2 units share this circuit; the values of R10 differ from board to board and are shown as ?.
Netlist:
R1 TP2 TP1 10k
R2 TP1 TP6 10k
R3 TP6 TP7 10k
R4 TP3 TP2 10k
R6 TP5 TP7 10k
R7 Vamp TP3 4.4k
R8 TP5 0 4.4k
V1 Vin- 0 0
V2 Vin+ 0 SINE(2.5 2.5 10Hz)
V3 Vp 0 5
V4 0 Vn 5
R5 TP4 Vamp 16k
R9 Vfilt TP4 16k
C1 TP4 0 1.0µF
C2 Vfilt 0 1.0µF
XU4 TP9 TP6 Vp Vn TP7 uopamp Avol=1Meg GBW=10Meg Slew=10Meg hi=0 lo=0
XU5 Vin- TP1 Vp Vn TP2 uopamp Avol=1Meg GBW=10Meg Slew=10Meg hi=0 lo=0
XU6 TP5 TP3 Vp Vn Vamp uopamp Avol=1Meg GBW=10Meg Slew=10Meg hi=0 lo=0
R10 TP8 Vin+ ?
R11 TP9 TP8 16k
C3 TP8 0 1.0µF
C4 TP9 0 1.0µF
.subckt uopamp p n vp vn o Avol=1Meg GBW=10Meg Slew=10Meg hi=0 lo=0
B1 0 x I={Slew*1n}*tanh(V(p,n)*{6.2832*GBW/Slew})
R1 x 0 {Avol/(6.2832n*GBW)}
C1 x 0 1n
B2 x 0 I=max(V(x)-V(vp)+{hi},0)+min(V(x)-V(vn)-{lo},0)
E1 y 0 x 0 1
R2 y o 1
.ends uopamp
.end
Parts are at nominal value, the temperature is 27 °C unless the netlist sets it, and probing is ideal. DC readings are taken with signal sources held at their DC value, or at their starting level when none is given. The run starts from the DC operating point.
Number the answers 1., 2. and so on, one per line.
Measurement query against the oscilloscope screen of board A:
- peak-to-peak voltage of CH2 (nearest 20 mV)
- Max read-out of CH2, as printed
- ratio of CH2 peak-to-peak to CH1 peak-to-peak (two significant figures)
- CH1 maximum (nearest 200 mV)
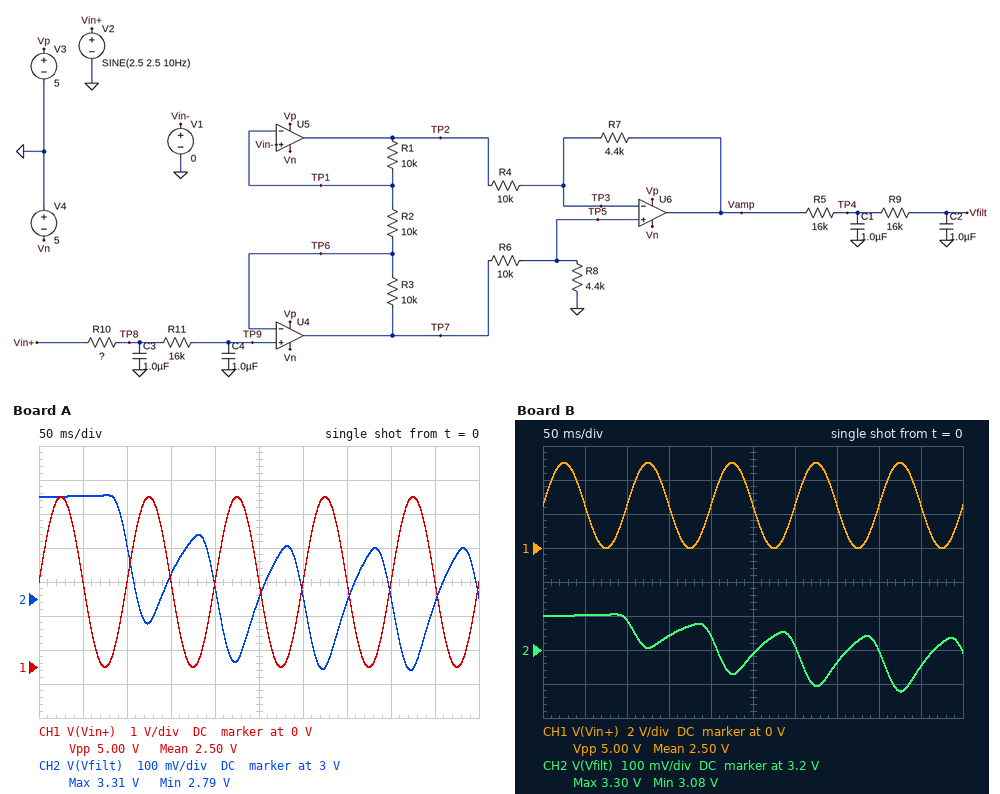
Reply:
1. 520 mV
2. 3.31 V
3. 0.10
4. 5.0 V
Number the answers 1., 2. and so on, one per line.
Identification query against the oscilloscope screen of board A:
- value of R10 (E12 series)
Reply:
1. 18 kΩ
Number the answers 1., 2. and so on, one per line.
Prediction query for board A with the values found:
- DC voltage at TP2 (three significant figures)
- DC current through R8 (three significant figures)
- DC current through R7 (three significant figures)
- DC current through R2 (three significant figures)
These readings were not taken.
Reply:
1. -2.50 V
2. 347 µA
3. 403 µA
4. 250 µA
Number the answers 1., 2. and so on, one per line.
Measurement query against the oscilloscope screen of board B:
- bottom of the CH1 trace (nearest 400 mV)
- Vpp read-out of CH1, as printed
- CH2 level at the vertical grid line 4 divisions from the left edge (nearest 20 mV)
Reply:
1. 0 V
2. 5.00 V
3. 3.24 V
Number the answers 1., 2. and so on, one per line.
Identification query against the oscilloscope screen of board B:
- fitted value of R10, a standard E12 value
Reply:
1. 47 kΩ
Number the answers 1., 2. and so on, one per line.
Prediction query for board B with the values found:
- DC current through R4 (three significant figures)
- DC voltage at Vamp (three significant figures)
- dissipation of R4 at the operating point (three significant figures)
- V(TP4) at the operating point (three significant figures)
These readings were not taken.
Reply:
1. 403 µA
2. 3.30 V
3. 1.62 mW
4. 3.30 V
